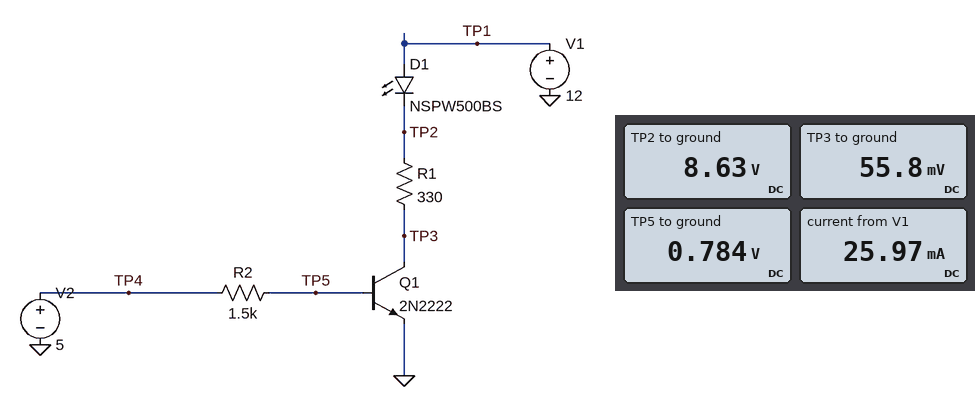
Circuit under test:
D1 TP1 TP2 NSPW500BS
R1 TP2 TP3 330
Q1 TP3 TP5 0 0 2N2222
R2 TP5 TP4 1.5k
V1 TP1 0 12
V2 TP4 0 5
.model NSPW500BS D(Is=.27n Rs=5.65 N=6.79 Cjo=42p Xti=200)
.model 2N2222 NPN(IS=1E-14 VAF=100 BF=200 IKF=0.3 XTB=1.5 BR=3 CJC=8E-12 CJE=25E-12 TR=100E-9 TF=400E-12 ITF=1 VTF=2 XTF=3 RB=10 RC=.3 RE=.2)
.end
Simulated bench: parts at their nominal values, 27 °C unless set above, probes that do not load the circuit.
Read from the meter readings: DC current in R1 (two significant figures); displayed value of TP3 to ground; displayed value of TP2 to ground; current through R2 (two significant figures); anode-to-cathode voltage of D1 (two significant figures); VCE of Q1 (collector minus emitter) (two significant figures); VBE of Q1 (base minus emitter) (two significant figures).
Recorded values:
26 mA
55.8 mV
8.63 V
2.8 mA
3.4 V
56 mV
780 mV
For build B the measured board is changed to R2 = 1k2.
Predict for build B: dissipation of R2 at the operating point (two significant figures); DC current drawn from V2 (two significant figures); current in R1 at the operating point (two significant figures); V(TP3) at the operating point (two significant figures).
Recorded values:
15 mW
3.5 mA
26 mA
52 mV
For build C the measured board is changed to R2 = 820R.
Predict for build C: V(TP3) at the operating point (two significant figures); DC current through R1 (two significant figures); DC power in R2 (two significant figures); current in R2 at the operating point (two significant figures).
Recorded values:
46 mV
26 mA
21 mW
5.1 mA
